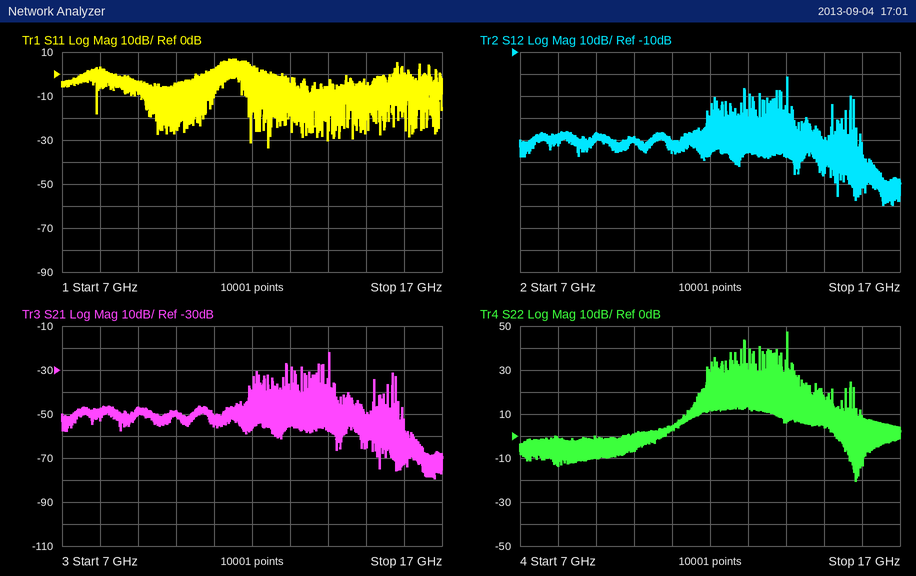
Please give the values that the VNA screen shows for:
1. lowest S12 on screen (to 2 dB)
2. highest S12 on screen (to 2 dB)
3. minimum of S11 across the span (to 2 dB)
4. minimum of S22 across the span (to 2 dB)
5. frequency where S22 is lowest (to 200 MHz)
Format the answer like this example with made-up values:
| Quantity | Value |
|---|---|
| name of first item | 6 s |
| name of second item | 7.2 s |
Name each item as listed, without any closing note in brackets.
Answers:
| Quantity | Value |
|---|---|
| lowest S12 on screen | -80 dB |
| highest S12 on screen | -22 dB |
| minimum of S11 across the span | -34 dB |
| minimum of S22 across the span | -20 dB |
| frequency where S22 is lowest | 15.8 GHz |
